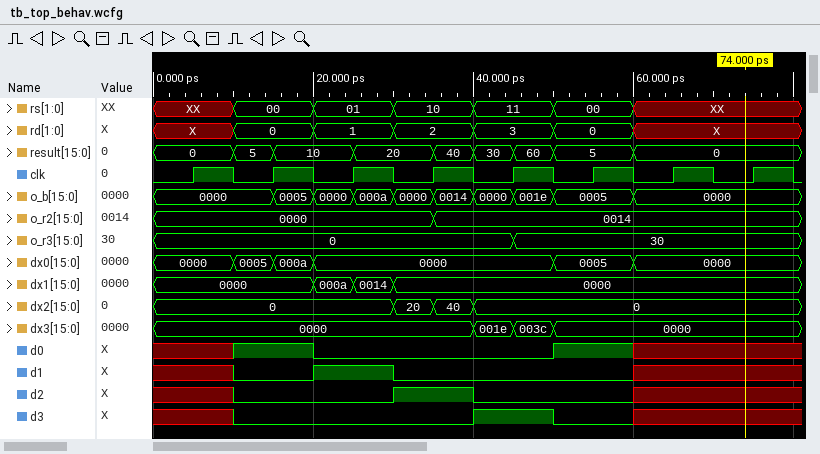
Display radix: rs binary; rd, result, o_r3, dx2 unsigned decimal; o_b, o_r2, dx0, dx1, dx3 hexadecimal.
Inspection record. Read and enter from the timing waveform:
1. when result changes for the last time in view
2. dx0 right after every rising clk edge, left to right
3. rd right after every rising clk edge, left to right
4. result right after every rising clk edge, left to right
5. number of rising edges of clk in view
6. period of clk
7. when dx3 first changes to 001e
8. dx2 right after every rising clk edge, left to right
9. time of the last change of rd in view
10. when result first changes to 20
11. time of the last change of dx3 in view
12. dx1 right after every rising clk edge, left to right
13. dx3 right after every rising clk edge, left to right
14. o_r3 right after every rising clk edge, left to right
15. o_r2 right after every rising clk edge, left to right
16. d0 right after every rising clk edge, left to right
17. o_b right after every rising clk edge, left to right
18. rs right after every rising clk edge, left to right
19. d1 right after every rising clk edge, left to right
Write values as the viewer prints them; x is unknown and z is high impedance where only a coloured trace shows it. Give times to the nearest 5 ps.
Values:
60 ps
0000, 000a, 0000, 0000, 0000, 0005, 0000, 0000
X, 0, 1, 2, 3, 0, X, X
0, 10, 20, 40, 60, 5, 0, 0
8
10 ps
40 ps
0, 0, 0, 40, 0, 0, 0, 0
60 ps
25 ps
50 ps
0000, 0000, 0014, 0000, 0000, 0000, 0000, 0000
0000, 0000, 0000, 0000, 003c, 0000, 0000, 0000
0, 0, 0, 0, 30, 30, 30, 30
0000, 0000, 0000, 0014, 0014, 0014, 0014, 0014
x 1 0 0 0 1 x x
0000, 0005, 000a, 0014, 001e, 0005, 0000, 0000
XX, 00, 01, 10, 11, 00, XX, XX
x 0 1 0 0 0 x x
